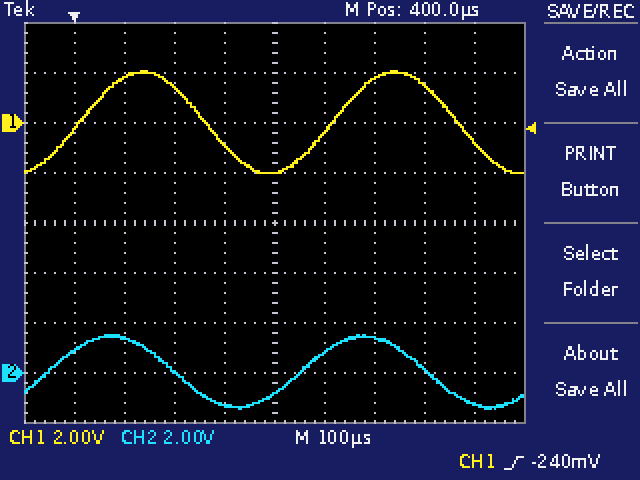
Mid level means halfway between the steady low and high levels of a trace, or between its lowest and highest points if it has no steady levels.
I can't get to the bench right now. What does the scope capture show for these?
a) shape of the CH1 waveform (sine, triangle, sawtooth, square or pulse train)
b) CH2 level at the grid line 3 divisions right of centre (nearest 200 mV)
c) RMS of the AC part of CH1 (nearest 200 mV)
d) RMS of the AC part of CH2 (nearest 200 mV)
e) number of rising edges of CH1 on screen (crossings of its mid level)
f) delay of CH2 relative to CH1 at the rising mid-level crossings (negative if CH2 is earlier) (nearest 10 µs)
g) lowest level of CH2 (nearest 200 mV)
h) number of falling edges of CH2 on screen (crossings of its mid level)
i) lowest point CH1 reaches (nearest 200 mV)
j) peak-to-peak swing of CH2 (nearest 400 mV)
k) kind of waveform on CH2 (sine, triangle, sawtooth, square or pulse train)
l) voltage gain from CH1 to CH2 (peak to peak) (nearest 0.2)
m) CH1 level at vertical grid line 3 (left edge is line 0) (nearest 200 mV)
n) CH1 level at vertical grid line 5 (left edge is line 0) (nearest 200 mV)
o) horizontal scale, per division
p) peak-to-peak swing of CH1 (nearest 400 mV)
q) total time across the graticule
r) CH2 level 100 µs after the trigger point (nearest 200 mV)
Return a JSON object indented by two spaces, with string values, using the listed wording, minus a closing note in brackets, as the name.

{
  "shape of the CH1 waveform": "sine",
  "CH2 level at the grid line 3 divisions right of centre": "200 mV",
  "RMS of the AC part of CH1": "1.4 V",
  "RMS of the AC part of CH2": "1.0 V",
  "number of rising edges of CH1 on screen": "2",
  "delay of CH2 relative to CH1 at the rising mid-level crossings (negative if CH2 is earlier)": "-60 µs",
  "lowest level of CH2": "-1.4 V",
  "number of falling edges of CH2 on screen": "2",
  "lowest point CH1 reaches": "-2.0 V",
  "peak-to-peak swing of CH2": "2.8 V",
  "kind of waveform on CH2": "sine",
  "voltage gain from CH1 to CH2 (peak to peak)": "0.8",
  "CH1 level at vertical grid line 3 (left edge is line 0)": "1.4 V",
  "CH1 level at vertical grid line 5 (left edge is line 0)": "-2.0 V",
  "horizontal scale, per division": "100 µs",
  "peak-to-peak swing of CH1": "4.0 V",
  "total time across the graticule": "1 ms",
  "CH2 level 100 µs after the trigger point": "1.4 V"
}
